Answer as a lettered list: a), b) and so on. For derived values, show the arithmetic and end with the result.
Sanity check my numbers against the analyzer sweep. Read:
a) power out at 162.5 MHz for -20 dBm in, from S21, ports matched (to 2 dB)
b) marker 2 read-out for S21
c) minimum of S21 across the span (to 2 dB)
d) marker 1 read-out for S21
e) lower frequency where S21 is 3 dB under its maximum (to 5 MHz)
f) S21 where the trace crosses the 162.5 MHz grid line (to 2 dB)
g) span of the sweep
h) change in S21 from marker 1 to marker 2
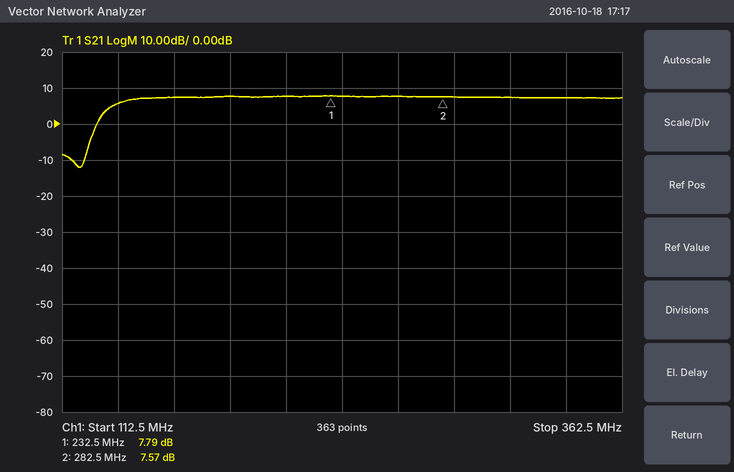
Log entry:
a) -20 dBm + (8 dB) = -12 dBm
b) 7.57 dB
c) -12 dB
d) 7.79 dB
e) 135 MHz
f) 8 dB
g) 250 MHz
h) 7.57 − (7.79) = -0.22 dB
